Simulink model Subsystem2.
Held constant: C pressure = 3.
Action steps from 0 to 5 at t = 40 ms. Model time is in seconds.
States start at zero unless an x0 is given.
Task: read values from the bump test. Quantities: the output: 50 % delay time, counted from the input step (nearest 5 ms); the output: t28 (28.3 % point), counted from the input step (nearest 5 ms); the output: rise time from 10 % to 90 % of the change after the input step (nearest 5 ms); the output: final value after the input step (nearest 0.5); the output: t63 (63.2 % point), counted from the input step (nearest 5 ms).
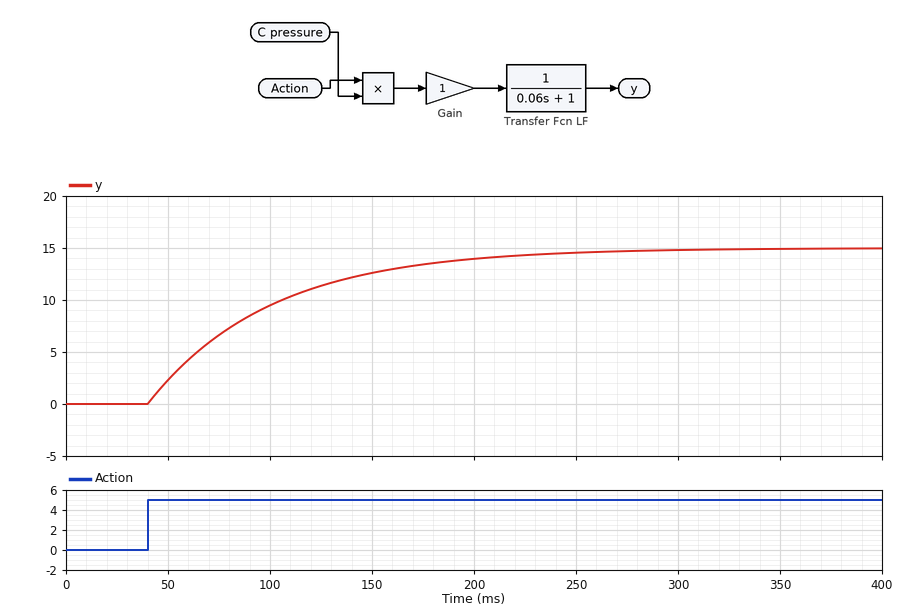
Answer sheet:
40 ms
20 ms
130 ms
15.0
60 ms
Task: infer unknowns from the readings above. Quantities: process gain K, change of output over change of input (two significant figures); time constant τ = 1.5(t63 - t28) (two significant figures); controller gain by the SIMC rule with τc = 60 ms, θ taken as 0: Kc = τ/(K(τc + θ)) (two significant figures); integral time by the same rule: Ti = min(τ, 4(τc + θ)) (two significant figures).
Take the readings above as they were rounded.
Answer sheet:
3.0
60 ms
0.33
60 ms
